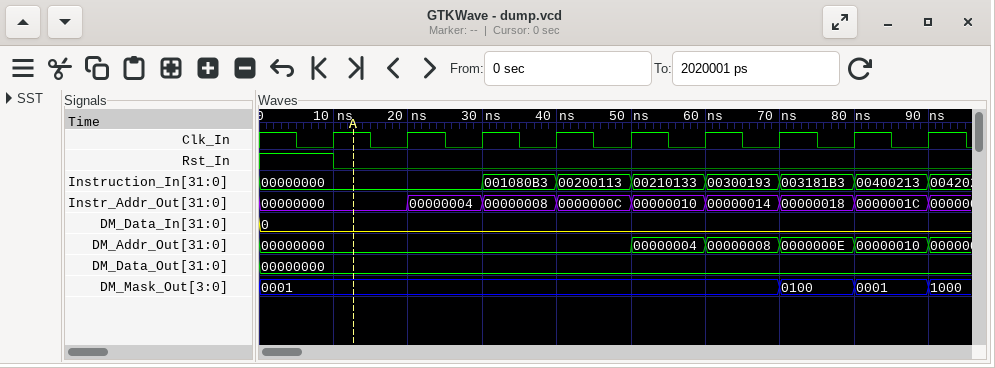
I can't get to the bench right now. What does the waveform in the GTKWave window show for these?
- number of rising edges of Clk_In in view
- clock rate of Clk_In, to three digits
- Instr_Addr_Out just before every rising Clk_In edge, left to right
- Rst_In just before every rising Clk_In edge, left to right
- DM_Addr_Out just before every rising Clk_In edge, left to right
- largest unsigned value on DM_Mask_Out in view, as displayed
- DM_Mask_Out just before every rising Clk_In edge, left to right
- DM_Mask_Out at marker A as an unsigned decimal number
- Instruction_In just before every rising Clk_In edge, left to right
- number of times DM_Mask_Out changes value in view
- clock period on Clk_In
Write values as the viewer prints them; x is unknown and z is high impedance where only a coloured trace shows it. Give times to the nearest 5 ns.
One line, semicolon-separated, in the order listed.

9; 100 MHz; 00000000, 00000000, 00000004, 00000008, 0000000C, 00000010, 00000014, 00000018, 0000001C; 1 0 0 0 0 0 0 0 0; 00000000, 00000000, 00000000, 00000000, 00000000, 00000004, 00000008, 0000000E, 00000010; 1000; 0001, 0001, 0001, 0001, 0001, 0001, 0001, 0100, 0001; 1; 00000000, 00000000, 00000000, 001080B3, 00200113, 00210133, 00300193, 003181B3, 00400213; 3; 10 ns
